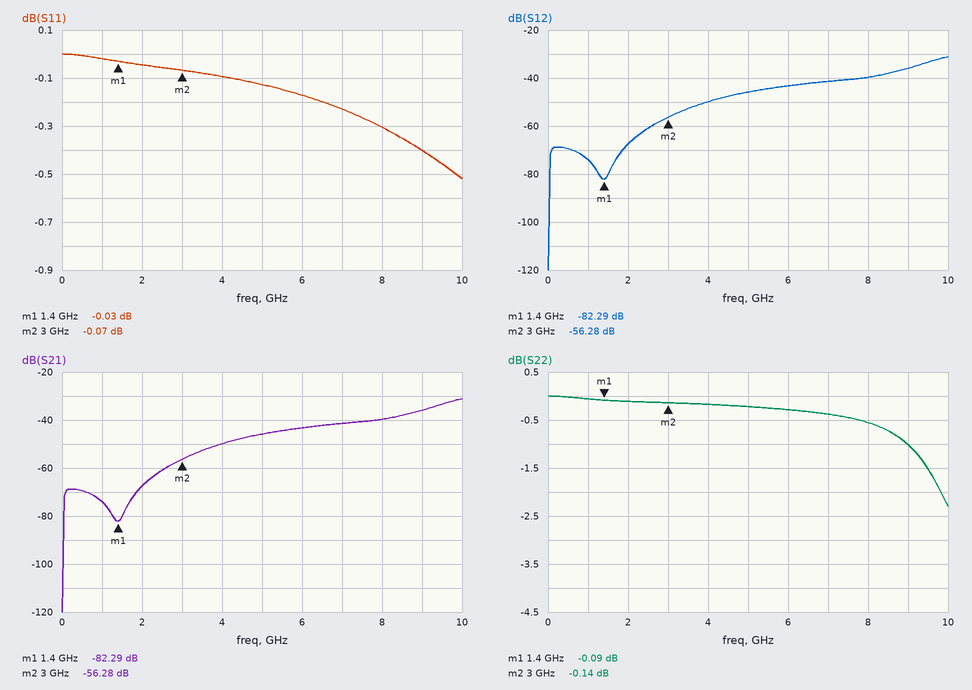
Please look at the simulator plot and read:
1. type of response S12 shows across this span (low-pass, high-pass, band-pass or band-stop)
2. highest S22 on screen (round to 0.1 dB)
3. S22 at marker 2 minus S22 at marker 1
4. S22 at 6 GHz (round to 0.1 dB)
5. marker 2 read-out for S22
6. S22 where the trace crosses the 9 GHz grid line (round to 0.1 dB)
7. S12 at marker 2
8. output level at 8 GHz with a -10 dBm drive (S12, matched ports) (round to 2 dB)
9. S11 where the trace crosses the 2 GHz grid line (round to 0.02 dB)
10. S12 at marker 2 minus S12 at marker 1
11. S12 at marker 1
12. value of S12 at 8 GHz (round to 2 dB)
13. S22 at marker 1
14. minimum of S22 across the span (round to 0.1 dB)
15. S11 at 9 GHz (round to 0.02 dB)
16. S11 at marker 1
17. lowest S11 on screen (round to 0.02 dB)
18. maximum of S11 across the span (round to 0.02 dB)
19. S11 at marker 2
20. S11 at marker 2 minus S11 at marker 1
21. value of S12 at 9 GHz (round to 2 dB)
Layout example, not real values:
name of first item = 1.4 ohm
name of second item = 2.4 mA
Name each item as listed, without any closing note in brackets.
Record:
type of response S12 shows across this span = high-pass
highest S22 on screen = 0.0 dB
S22 at marker 2 minus S22 at marker 1 = -0.05 dB
S22 at 6 GHz = -0.3 dB
marker 2 read-out for S22 = -0.14 dB
S22 where the trace crosses the 9 GHz grid line = -1.0 dB
S12 at marker 2 = -56.28 dB
output level at 8 GHz with a -10 dBm drive (S12, matched ports) = -50 dBm
S11 where the trace crosses the 2 GHz grid line = -0.04 dB
S12 at marker 2 minus S12 at marker 1 = 26.01 dB
S12 at marker 1 = -82.29 dB
value of S12 at 8 GHz = -40 dB
S22 at marker 1 = -0.09 dB
minimum of S22 across the span = -2.3 dB
S11 at 9 GHz = -0.40 dB
S11 at marker 1 = -0.03 dB
lowest S11 on screen = -0.52 dB
maximum of S11 across the span = 0.00 dB
S11 at marker 2 = -0.07 dB
S11 at marker 2 minus S11 at marker 1 = -0.04 dB
value of S12 at 9 GHz = -36 dB
